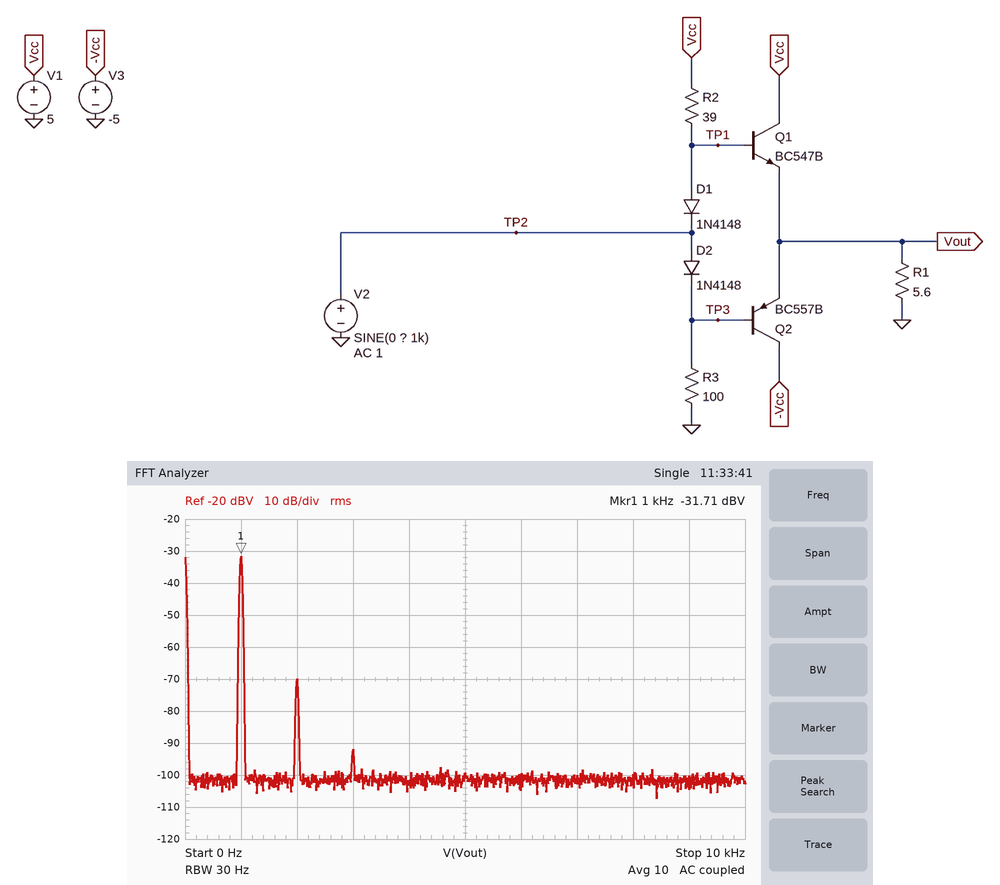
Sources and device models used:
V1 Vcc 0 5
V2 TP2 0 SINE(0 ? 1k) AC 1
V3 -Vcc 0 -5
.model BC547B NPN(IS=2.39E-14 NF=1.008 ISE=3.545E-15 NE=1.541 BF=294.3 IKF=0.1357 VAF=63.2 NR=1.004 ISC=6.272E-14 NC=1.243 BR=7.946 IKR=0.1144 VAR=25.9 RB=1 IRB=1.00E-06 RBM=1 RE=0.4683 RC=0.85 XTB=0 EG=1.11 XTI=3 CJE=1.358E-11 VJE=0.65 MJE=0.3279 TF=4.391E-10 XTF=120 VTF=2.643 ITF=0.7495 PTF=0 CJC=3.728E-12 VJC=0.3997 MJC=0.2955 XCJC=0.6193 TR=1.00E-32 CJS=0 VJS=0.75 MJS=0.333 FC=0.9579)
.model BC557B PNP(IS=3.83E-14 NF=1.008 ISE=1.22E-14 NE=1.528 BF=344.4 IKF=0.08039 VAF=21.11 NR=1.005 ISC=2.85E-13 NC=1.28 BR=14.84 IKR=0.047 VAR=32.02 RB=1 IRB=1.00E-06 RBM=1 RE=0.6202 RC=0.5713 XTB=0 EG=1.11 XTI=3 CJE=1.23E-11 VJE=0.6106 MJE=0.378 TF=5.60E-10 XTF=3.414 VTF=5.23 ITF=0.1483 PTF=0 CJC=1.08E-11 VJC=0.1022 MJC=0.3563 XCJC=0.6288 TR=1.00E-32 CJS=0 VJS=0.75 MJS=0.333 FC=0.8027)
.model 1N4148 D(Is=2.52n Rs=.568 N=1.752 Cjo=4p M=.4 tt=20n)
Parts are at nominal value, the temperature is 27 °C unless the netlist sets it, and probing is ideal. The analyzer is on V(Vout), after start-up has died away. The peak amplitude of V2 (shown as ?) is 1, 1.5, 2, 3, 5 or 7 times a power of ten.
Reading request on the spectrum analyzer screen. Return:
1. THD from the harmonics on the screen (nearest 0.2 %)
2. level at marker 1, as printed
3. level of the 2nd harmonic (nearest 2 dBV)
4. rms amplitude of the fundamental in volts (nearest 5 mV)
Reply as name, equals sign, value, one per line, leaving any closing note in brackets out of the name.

THD from the harmonics on the screen = 1.2 %
level at marker 1, as printed = -31.71 dBV
level of the 2nd harmonic = -70 dBV
rms amplitude of the fundamental in volts = 25 mV
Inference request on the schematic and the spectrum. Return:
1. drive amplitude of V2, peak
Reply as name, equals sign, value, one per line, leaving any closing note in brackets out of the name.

drive amplitude of V2, peak = 50 mV
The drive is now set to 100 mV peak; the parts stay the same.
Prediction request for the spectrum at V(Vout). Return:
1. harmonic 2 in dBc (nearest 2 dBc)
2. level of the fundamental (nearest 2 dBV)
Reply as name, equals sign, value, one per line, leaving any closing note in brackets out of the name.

harmonic 2 in dBc = -32 dBc
level of the fundamental = -26 dBV
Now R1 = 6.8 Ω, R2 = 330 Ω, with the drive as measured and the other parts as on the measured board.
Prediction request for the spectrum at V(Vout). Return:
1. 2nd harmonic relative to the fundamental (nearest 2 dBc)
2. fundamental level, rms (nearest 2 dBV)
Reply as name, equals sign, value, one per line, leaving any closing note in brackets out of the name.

2nd harmonic relative to the fundamental = -20 dBc
fundamental level, rms = -36 dBV
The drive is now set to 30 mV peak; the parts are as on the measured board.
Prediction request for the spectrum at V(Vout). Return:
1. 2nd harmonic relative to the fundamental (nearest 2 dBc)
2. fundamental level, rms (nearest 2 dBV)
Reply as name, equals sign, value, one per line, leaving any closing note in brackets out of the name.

2nd harmonic relative to the fundamental = -42 dBc
fundamental level, rms = -36 dBV
